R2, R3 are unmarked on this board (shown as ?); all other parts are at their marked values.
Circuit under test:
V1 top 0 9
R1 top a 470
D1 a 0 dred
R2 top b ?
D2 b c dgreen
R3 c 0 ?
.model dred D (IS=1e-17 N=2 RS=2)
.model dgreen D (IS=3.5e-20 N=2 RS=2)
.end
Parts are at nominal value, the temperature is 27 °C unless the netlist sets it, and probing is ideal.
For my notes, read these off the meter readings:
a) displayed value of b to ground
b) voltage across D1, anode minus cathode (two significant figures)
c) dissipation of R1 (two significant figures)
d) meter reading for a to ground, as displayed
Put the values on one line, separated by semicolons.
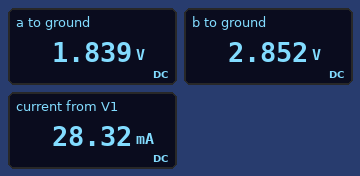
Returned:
2.852 V; 1.8 V; 110 mW; 1.839 V
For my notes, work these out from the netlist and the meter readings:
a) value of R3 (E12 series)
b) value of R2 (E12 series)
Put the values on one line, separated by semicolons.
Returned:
56 Ω; 470 Ω
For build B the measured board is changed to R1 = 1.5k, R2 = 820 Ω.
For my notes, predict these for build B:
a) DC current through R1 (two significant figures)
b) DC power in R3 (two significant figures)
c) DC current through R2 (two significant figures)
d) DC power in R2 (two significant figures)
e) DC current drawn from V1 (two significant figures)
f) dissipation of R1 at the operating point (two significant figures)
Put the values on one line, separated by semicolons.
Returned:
4.8 mA; 3.5 mW; 7.9 mA; 51 mW; 13 mA; 35 mW
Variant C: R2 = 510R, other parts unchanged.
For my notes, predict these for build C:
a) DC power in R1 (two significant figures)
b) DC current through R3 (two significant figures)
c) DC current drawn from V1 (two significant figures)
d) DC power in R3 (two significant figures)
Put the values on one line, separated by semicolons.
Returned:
110 mW; 12 mA; 27 mA; 8.3 mW
